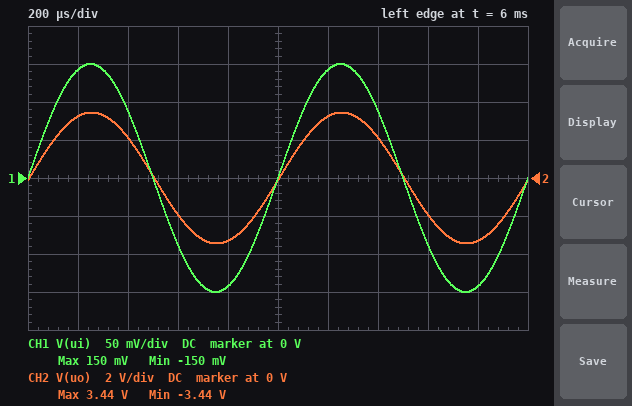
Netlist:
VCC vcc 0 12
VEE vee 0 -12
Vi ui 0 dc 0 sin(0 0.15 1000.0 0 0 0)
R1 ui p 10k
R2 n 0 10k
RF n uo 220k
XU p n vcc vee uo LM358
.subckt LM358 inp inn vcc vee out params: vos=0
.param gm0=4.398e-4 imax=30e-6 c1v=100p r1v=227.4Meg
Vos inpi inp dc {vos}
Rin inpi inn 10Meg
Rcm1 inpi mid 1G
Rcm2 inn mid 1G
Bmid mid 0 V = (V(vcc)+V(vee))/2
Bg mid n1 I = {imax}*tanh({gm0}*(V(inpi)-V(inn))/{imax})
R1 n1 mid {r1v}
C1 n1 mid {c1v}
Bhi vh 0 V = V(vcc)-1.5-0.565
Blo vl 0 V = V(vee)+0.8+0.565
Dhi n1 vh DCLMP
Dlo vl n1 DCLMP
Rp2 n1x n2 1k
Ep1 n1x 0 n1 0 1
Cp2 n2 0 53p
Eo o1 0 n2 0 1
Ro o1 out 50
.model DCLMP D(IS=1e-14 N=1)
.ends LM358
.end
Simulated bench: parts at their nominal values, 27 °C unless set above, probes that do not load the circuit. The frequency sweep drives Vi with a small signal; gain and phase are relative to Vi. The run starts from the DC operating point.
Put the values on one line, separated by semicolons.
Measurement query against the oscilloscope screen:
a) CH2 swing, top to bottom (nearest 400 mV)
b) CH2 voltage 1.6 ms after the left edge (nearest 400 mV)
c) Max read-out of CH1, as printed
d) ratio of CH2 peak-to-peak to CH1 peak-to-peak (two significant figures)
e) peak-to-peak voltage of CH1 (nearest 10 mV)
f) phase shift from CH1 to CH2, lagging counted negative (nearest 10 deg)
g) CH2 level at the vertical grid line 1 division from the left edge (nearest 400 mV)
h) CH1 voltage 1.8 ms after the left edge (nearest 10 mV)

6.8 V; -2.0 V; 150 mV; 23; 300 mV; 0 deg; 3.2 V; -140 mV
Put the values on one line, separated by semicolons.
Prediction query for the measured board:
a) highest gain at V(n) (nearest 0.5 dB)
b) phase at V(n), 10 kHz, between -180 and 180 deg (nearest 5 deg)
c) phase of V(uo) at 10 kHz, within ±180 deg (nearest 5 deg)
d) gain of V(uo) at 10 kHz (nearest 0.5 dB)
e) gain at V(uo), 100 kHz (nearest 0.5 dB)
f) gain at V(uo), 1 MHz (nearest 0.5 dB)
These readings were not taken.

0 dB; -20 deg; -20 deg; 27.0 dB; 16.5 dB; -3.5 dB
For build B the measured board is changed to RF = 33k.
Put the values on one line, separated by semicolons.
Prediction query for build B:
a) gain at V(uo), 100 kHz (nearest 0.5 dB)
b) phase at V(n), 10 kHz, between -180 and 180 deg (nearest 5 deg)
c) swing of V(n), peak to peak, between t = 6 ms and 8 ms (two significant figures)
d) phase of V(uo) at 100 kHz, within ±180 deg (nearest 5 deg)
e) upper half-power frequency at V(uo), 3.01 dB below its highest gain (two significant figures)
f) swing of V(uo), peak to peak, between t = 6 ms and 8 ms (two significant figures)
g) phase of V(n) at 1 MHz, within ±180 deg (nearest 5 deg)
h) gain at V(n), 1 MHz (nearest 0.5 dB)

11.5 dB; -5 deg; 300 mV; -30 deg; 170 kHz; 1.3 V; -100 deg; -16.0 dB
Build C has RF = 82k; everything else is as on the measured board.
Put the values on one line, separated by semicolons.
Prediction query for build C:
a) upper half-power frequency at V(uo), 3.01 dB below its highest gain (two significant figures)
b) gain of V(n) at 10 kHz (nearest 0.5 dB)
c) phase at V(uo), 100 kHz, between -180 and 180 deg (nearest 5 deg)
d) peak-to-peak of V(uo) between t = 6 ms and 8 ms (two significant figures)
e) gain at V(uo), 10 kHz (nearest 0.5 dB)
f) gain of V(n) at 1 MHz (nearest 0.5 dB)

78 kHz; 0 dB; -55 deg; 2.8 V; 19.0 dB; -22.5 dB
